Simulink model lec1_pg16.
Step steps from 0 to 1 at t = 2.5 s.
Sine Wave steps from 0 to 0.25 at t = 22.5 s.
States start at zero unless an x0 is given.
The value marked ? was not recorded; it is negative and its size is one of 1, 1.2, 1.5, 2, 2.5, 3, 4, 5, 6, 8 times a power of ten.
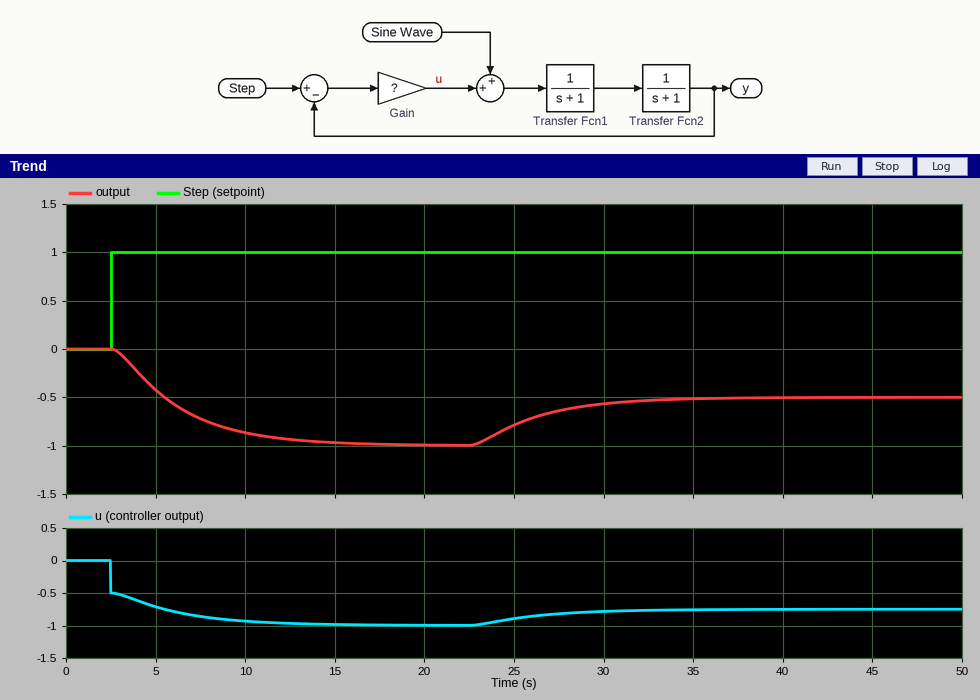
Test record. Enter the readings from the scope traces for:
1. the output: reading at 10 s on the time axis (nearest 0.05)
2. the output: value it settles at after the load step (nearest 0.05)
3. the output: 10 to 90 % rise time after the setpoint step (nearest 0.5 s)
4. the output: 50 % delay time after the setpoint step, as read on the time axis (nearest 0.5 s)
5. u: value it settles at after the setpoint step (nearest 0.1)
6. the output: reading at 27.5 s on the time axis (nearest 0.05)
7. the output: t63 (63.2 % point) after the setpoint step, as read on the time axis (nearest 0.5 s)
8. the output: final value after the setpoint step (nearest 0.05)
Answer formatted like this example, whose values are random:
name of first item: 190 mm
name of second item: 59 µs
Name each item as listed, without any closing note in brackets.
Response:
the output: reading at 10 s on the time axis: -0.85
the output: value it settles at after the load step: -0.50
the output: 10 to 90 % rise time after the setpoint step: 7.5 s
the output: 50 % delay time after the setpoint step, as read on the time axis: 5.5 s
u: value it settles at after the setpoint step: -1.0
the output: reading at 27.5 s on the time axis: -0.65
the output: t63 (63.2 % point) after the setpoint step, as read on the time axis: 6.5 s
the output: final value after the setpoint step: -1.00
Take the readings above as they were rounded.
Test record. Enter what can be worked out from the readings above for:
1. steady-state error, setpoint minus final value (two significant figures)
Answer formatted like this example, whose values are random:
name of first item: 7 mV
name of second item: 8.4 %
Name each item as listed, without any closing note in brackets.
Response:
steady-state error, setpoint minus final value: 2.0
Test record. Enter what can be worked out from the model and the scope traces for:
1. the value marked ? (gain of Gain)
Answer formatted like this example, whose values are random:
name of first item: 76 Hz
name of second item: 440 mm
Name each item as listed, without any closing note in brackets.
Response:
the value marked ?: -0.5
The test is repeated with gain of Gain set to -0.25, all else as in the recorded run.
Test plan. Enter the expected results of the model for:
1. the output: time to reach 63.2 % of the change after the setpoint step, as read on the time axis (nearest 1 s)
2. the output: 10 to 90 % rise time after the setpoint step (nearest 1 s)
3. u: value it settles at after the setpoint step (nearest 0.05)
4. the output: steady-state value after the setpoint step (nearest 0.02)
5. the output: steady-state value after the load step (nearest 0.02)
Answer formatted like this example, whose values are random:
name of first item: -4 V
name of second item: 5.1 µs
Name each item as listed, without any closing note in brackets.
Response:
the output: time to reach 63.2 % of the change after the setpoint step, as read on the time axis: 5 s
the output: 10 to 90 % rise time after the setpoint step: 5 s
u: value it settles at after the setpoint step: -0.35
the output: steady-state value after the setpoint step: -0.34
the output: steady-state value after the load step: 0.00
